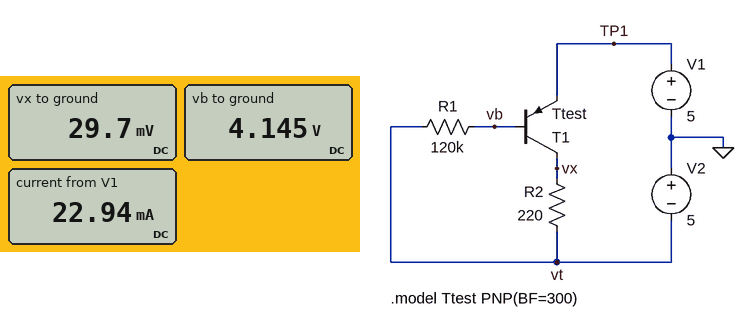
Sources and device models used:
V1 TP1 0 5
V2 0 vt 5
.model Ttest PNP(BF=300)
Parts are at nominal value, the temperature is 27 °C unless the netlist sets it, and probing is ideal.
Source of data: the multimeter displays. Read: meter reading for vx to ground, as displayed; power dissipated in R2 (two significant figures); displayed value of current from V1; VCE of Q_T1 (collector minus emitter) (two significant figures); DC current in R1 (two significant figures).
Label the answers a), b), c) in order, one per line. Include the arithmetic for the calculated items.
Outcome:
a) 29.7 mV
b) (29.7 mV - (-5 V))^2 / 220 Ω = 110 mW
c) 22.94 mA
d) 29.7 mV - 5 V = -5.0 V
e) (4.145 V - (-5 V)) / 120 kΩ = 76 µA
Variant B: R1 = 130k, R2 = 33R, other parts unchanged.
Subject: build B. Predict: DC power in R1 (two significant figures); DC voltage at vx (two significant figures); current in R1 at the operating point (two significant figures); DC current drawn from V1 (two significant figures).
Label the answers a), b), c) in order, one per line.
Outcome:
a) 640 µW
b) -4.3 V
c) 70 µA
d) 21 mA
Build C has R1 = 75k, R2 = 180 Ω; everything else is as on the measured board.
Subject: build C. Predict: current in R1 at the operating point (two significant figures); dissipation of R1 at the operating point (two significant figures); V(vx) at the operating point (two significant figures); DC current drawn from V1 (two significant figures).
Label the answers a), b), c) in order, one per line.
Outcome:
a) 120 µA
b) 1.1 mW
c) 1.6 V
d) 37 mA
